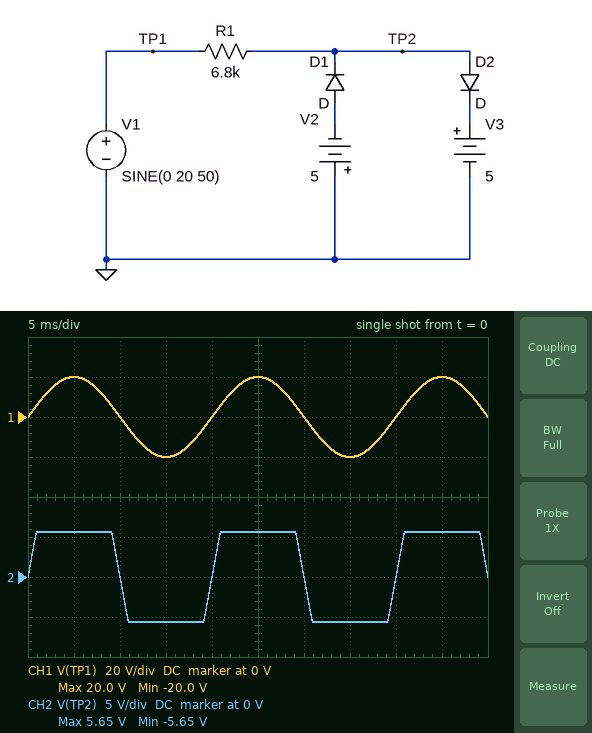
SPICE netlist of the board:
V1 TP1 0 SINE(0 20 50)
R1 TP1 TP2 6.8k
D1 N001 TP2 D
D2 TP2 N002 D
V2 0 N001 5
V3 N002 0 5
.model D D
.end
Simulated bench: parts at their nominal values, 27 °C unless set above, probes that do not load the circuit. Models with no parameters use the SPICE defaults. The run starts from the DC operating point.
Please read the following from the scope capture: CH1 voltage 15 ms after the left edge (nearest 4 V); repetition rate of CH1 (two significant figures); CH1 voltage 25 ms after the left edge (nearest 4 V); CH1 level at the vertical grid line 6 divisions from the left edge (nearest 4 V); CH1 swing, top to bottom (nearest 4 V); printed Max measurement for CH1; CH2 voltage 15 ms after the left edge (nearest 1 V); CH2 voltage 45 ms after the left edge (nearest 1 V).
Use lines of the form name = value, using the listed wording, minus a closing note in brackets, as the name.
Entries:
CH1 voltage 15 ms after the left edge = -20 V
repetition rate of CH1 = 50 Hz
CH1 voltage 25 ms after the left edge = 20 V
CH1 level at the vertical grid line 6 divisions from the left edge = 0 V
CH1 swing, top to bottom = 40 V
printed Max measurement for CH1 = 20.0 V
CH2 voltage 15 ms after the left edge = -6 V
CH2 voltage 45 ms after the left edge = 6 V
